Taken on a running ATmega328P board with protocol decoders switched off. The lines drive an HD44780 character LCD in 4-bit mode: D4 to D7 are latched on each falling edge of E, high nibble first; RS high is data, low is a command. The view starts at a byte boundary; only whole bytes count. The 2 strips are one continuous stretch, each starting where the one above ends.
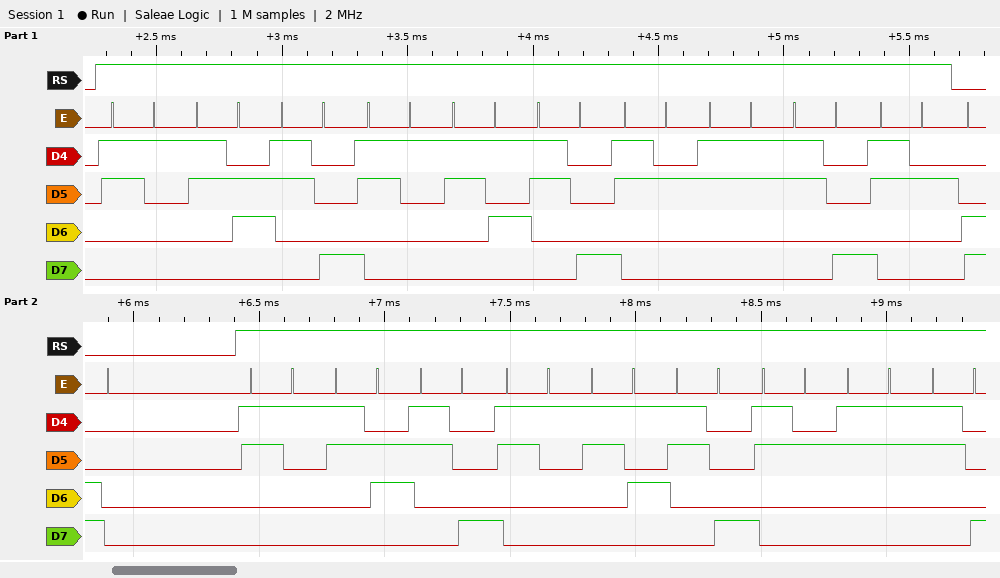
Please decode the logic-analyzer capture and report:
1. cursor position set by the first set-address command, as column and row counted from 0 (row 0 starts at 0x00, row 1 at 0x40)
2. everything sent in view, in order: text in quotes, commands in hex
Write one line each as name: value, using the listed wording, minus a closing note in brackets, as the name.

cursor position set by the first set-address command, as column and row counted from 0: column 0, row 1
everything sent in view, in order: text in quotes, commands in hex: "1681582382" 0xC0 "168158238"
